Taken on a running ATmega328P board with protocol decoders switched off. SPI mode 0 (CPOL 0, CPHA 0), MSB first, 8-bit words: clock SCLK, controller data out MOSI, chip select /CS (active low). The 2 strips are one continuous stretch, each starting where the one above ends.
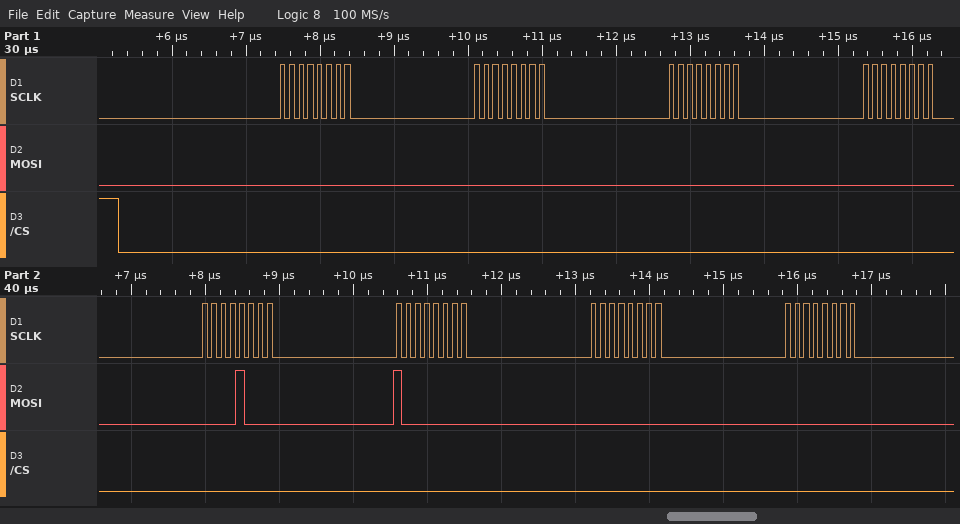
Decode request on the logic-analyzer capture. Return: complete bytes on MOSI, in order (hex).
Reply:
00 00 00 00 08 80 00 00
